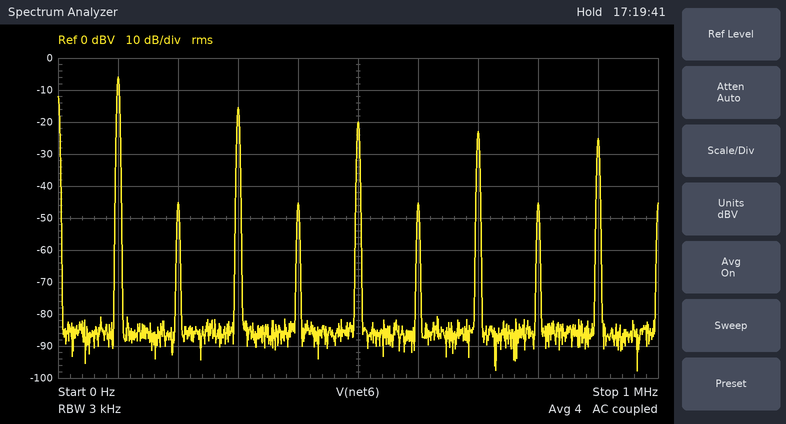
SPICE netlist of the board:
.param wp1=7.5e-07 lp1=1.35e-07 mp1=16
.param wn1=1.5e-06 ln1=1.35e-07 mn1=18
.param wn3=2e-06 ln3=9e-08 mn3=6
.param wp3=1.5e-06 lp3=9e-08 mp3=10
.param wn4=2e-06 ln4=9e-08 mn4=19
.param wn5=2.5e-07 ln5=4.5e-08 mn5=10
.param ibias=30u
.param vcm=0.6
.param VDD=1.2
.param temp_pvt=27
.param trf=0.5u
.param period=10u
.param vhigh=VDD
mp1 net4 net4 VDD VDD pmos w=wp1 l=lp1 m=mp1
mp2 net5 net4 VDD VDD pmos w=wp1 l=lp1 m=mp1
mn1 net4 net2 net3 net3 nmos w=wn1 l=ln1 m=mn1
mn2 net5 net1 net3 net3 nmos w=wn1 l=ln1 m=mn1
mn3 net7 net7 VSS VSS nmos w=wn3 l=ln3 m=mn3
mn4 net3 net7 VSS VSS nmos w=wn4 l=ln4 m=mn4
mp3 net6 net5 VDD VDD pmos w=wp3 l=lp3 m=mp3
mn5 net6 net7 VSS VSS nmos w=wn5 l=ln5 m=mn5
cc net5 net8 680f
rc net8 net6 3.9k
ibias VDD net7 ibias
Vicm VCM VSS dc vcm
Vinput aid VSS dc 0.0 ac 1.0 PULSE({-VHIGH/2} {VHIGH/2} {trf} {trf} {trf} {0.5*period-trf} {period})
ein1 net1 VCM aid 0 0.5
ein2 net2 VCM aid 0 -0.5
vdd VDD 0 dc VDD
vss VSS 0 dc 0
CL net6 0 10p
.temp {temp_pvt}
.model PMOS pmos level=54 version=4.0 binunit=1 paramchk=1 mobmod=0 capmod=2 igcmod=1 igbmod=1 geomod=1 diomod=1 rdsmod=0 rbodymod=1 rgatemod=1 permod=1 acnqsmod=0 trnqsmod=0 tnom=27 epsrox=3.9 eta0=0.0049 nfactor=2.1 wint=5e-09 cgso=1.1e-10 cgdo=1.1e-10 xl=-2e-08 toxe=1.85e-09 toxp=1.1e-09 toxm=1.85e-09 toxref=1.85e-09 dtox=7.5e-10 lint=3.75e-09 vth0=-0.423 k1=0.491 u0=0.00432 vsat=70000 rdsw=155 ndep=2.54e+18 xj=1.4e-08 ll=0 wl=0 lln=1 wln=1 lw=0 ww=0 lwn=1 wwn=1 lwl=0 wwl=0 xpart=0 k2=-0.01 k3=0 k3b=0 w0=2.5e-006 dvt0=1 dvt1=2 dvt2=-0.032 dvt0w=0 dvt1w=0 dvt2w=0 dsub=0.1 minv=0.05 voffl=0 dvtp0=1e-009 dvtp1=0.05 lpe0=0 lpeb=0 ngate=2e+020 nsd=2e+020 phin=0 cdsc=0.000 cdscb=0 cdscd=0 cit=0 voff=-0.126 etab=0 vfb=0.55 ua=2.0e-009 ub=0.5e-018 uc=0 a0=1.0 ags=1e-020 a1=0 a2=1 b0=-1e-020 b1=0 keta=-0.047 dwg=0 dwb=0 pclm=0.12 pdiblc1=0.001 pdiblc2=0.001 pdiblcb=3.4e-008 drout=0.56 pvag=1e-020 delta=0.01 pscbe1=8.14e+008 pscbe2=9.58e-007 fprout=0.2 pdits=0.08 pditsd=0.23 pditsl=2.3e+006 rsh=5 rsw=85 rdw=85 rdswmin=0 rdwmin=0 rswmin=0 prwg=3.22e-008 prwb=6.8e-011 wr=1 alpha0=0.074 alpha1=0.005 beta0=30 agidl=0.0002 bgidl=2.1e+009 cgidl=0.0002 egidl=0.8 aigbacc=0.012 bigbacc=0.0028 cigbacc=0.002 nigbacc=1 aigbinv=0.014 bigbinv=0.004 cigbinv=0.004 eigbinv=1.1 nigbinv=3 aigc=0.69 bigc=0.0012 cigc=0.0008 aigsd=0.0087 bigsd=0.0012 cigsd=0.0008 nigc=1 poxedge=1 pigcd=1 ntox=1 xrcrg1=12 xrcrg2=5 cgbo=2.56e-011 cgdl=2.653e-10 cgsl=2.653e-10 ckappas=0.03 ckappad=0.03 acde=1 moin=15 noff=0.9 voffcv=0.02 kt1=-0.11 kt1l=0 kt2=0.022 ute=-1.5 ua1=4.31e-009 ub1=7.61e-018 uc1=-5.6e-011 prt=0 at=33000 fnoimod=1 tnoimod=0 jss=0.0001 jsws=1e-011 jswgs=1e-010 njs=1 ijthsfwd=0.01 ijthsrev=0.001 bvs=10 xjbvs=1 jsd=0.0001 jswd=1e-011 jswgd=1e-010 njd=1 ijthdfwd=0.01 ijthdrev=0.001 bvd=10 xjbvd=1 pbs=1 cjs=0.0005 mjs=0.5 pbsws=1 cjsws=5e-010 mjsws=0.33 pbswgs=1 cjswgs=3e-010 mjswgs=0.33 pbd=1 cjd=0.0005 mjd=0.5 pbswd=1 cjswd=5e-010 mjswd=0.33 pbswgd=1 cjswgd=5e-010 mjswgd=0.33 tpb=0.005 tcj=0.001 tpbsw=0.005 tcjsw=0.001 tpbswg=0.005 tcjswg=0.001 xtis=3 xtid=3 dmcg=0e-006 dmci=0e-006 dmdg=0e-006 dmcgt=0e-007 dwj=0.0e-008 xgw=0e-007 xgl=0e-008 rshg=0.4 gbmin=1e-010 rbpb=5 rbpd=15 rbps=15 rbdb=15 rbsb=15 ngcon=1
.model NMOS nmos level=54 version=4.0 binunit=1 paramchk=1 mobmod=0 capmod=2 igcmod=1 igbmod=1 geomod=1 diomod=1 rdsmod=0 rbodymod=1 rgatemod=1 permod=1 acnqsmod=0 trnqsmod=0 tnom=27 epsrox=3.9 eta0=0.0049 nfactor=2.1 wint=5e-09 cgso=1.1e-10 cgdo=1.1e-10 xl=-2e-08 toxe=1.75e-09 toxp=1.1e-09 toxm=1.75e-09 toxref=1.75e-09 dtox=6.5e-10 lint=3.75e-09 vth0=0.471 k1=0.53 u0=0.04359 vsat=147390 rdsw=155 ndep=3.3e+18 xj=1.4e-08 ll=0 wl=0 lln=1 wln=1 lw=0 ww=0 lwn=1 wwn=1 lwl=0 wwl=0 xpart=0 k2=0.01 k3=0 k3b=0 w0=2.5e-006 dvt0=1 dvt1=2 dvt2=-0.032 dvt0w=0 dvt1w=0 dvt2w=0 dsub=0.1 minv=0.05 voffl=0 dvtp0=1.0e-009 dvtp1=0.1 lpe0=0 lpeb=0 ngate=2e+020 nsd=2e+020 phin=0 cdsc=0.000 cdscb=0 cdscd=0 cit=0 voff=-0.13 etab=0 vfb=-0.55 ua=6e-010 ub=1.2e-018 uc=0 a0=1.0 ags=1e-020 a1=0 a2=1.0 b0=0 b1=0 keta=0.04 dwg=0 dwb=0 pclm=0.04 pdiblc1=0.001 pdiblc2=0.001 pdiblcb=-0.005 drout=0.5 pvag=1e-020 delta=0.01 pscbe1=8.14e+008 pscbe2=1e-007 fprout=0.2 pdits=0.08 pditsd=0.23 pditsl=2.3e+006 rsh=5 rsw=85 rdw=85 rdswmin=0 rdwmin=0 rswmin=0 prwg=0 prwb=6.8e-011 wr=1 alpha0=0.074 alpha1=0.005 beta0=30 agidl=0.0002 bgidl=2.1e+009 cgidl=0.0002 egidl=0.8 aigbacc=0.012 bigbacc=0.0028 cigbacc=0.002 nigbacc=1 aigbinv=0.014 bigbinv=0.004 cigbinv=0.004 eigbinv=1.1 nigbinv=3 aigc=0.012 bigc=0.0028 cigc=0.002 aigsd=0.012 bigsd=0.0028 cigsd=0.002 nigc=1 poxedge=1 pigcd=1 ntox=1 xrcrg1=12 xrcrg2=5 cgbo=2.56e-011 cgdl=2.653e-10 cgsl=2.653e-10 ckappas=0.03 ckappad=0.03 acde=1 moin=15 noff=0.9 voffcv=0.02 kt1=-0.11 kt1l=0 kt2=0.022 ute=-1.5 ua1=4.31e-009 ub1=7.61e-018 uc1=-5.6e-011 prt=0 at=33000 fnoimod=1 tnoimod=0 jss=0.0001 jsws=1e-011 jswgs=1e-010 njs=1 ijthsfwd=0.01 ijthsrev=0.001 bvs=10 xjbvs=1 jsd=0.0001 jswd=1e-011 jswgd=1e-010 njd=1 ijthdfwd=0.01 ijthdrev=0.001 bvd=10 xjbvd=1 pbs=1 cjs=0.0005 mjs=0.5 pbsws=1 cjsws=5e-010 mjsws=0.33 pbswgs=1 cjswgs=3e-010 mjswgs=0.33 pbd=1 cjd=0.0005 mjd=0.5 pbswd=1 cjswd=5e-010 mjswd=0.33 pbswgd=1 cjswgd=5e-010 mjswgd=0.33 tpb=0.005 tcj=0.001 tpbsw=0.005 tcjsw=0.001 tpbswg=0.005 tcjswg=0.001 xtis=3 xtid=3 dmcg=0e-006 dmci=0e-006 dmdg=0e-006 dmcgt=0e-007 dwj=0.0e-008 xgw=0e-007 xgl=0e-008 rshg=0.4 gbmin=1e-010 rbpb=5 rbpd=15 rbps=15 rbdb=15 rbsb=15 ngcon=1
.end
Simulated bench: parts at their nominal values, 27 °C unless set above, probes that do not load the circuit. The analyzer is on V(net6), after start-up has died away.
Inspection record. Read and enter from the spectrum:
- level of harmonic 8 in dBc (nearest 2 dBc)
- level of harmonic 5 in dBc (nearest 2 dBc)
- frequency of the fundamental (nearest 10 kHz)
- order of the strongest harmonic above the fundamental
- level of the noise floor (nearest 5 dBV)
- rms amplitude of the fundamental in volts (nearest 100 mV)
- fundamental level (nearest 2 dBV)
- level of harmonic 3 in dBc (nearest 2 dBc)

-40 dBc
-14 dBc
100 kHz
3
-85 dBV
500 mV
-6 dBV
-10 dBc
